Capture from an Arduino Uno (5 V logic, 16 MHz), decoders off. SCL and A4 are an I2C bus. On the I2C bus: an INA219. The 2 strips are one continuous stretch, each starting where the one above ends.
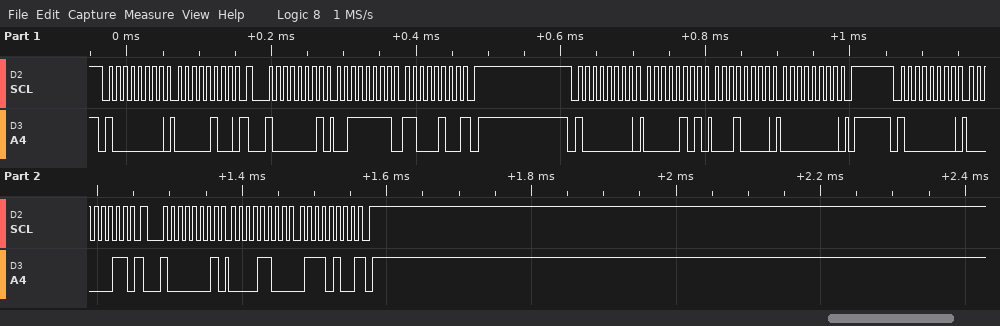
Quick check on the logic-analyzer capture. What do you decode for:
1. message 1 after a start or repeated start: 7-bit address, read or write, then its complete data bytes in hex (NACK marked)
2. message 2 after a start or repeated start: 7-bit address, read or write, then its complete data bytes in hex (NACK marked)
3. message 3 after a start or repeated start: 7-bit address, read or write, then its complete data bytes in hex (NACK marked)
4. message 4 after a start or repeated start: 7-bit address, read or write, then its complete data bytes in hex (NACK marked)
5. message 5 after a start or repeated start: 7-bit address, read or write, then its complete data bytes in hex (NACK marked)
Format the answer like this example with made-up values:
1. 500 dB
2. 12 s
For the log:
1. 0x40 write: 04
2. 0x40 read: 3F C4 NACK
3. 0x40 write: 05 10 00
4. 0x40 write: 03
5. 0x40 read: 0C 74 NACK
